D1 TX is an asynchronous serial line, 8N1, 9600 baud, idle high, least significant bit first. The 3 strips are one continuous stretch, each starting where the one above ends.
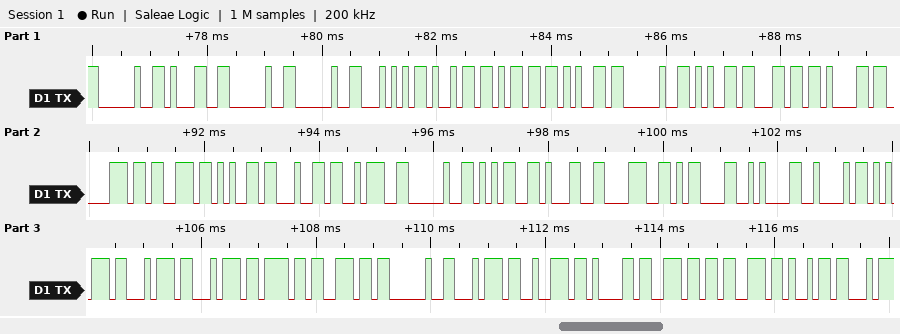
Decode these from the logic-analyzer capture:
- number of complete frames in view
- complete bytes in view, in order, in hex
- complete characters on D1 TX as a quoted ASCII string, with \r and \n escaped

36
0x20 0x31 0x20 0x20 0x54 0x69 0x6D 0x65 0x20 0x65 0x6C 0x61 0x70 0x73 0x65 0x64 0x3A 0x20 0x35 0x31 0x38 0x0D 0x0A 0x42 0x75 0x74 0x74 0x6F 0x6E 0x20 0x74 0x72 0x61 0x6E 0x73 0x69
" 1  Time elapsed: 518\r\nButton transi"
